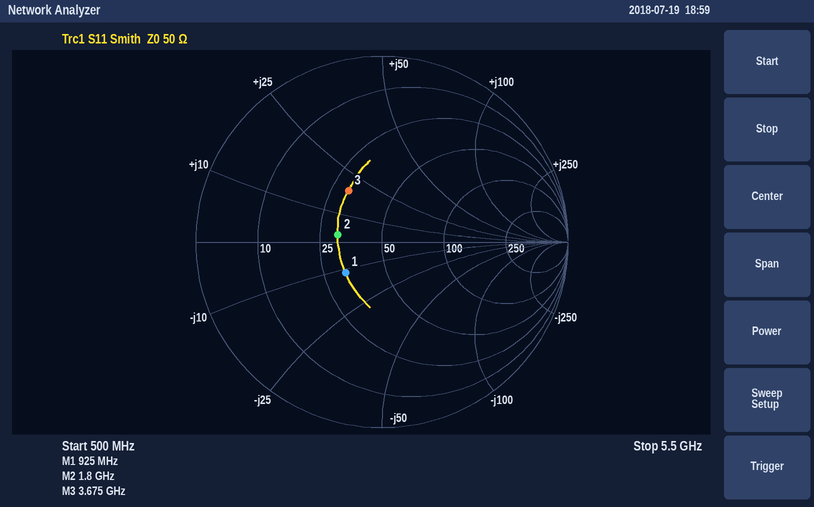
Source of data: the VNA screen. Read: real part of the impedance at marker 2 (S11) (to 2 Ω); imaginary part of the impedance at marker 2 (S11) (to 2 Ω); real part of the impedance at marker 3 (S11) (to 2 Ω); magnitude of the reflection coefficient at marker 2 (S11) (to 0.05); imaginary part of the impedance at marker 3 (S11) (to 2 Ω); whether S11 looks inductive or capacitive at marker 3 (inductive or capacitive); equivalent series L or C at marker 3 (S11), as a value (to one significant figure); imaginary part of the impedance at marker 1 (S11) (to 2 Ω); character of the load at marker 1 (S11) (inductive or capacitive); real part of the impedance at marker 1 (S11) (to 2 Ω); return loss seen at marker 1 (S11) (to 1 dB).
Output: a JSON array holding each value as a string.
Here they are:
["30 Ω", "+2 Ω", "30 Ω", "0.25", "+18 Ω", "inductive", "800 pH", "-12 Ω", "capacitive", "32 Ω", "12 dB"]
